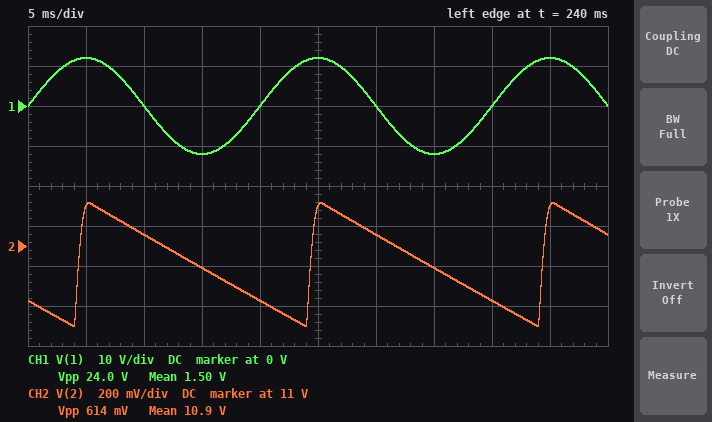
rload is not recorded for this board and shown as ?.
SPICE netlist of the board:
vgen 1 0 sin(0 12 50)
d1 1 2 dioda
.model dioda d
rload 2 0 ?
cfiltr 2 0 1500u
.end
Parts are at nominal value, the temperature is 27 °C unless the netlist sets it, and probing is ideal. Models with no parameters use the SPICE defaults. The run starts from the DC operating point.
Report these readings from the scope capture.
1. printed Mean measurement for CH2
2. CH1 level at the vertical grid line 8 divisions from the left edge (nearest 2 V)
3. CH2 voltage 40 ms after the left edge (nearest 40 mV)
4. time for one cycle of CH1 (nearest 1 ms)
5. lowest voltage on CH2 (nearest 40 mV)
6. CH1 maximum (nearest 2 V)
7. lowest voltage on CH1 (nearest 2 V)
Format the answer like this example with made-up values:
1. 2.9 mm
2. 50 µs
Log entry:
1. 10.9 V
2. 0 V
3. 10.72 V
4. 20 ms
5. 10.60 V
6. 12 V
7. -12 V
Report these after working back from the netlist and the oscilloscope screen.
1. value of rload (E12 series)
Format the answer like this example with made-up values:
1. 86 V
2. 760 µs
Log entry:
1. 220 Ω
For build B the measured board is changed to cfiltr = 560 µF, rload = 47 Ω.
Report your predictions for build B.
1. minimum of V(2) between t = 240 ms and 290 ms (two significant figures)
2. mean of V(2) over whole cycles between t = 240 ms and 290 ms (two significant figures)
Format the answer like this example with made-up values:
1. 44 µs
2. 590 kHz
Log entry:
1. 6.0 V
2. 8.5 V
